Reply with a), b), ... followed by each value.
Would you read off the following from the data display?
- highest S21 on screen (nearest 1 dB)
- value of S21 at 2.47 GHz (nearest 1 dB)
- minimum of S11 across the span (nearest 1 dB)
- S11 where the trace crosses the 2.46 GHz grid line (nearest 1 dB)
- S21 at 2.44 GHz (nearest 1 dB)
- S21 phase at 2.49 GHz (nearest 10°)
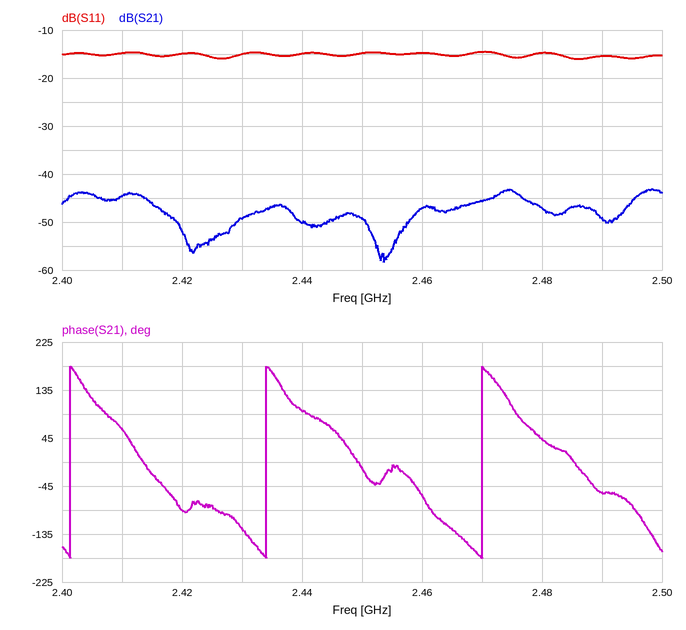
a) -43 dB
b) -46 dB
c) -16 dB
d) -15 dB
e) -50 dB
f) -60°
